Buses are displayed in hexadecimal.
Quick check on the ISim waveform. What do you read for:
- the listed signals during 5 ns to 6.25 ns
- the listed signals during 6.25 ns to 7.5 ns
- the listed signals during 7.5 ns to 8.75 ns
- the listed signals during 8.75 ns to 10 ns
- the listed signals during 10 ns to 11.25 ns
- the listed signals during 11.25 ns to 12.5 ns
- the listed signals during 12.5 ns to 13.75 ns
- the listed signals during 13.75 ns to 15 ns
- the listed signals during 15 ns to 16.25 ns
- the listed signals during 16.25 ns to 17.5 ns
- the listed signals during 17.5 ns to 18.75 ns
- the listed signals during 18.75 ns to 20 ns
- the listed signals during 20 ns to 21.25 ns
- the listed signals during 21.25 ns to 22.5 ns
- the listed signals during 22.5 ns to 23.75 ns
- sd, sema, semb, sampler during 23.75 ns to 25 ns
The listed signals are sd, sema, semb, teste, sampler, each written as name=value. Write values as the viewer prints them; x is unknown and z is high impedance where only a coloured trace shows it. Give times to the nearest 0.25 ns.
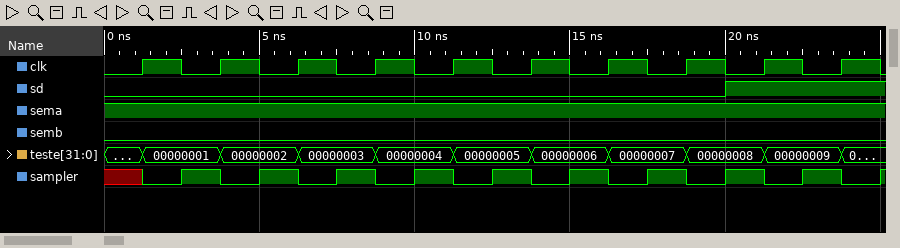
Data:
sd=0, sema=1, semb=0, teste=00000002, sampler=1
sd=0, sema=1, semb=0, teste=00000003, sampler=0
sd=0, sema=1, semb=0, teste=00000003, sampler=1
sd=0, sema=1, semb=0, teste=00000004, sampler=0
sd=0, sema=1, semb=0, teste=00000004, sampler=1
sd=0, sema=1, semb=0, teste=00000005, sampler=0
sd=0, sema=1, semb=0, teste=00000005, sampler=1
sd=0, sema=1, semb=0, teste=00000006, sampler=0
sd=0, sema=1, semb=0, teste=00000006, sampler=1
sd=0, sema=1, semb=0, teste=00000007, sampler=0
sd=0, sema=1, semb=0, teste=00000007, sampler=1
sd=0, sema=1, semb=0, teste=00000008, sampler=0
sd=1, sema=1, semb=0, teste=00000008, sampler=1
sd=1, sema=1, semb=0, teste=00000009, sampler=0
sd=1, sema=1, semb=0, teste=00000009, sampler=1
sd=1, sema=1, semb=0, sampler=0
